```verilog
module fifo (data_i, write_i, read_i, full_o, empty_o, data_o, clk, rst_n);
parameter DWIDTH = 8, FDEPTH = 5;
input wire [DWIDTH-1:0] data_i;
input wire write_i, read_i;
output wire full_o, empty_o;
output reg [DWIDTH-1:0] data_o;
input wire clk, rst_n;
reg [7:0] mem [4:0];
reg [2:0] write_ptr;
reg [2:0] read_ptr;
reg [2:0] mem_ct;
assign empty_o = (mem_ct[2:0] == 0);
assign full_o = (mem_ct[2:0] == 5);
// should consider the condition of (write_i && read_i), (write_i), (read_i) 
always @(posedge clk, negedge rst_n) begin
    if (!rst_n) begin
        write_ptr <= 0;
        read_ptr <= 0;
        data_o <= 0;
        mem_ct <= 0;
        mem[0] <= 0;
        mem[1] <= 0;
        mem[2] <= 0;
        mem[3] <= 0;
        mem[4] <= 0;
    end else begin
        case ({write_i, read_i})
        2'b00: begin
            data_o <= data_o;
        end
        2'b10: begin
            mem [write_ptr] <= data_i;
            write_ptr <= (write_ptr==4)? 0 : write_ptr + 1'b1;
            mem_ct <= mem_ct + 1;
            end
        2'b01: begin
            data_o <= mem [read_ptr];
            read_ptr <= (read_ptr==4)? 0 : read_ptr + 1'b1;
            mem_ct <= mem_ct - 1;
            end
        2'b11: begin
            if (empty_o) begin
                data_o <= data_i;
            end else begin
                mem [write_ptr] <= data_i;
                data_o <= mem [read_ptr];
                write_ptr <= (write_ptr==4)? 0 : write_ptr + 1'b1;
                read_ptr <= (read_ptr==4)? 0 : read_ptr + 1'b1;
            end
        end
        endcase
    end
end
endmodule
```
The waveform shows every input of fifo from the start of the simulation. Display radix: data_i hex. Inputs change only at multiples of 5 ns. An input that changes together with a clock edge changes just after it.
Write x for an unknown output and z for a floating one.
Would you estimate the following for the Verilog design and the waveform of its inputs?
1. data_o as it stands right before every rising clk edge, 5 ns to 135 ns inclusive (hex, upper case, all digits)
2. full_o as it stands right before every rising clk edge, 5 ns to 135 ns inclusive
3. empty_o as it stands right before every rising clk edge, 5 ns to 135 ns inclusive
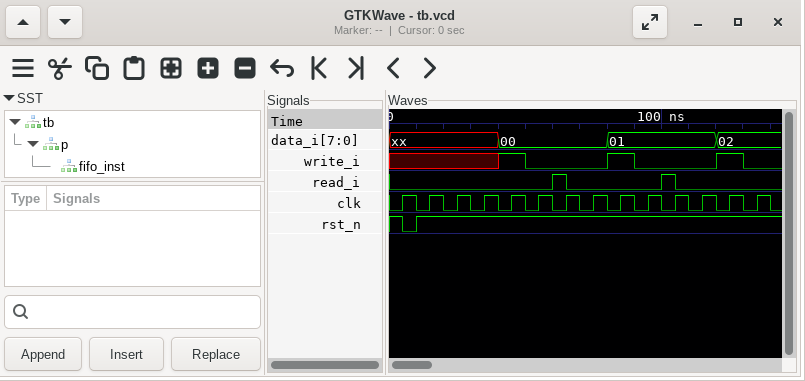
x, 00, 00, 00, 00, 00, 00, 00, 00, 00, 00, 01, 01, 01
x 0 0 0 0 0 0 0 0 0 0 0 0 0
x 1 1 1 1 0 0 1 1 0 0 1 1 0
